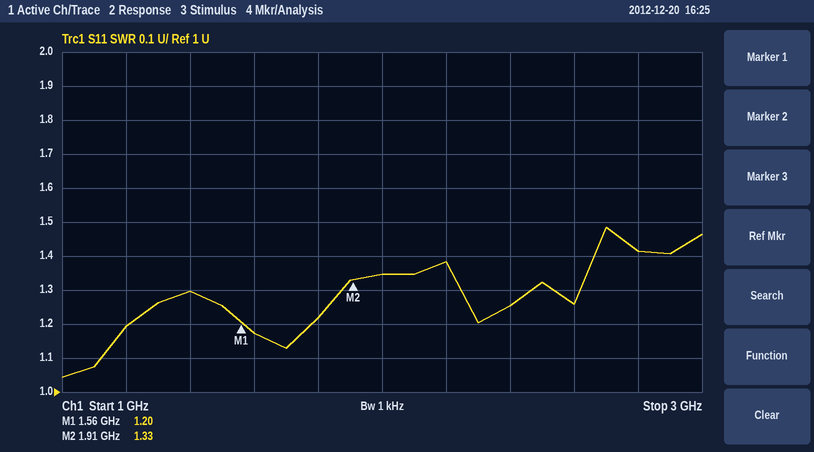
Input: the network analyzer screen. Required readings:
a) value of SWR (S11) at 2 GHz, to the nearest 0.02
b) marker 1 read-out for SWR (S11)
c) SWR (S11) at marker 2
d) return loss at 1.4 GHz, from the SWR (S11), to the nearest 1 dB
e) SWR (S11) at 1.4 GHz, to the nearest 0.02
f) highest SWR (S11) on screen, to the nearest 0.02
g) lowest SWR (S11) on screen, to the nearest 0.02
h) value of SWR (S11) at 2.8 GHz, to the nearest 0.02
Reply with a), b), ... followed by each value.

a) 1.34
b) 1.20
c) 1.33
d) 18 dB
e) 1.30
f) 1.48
g) 1.04
h) 1.42
